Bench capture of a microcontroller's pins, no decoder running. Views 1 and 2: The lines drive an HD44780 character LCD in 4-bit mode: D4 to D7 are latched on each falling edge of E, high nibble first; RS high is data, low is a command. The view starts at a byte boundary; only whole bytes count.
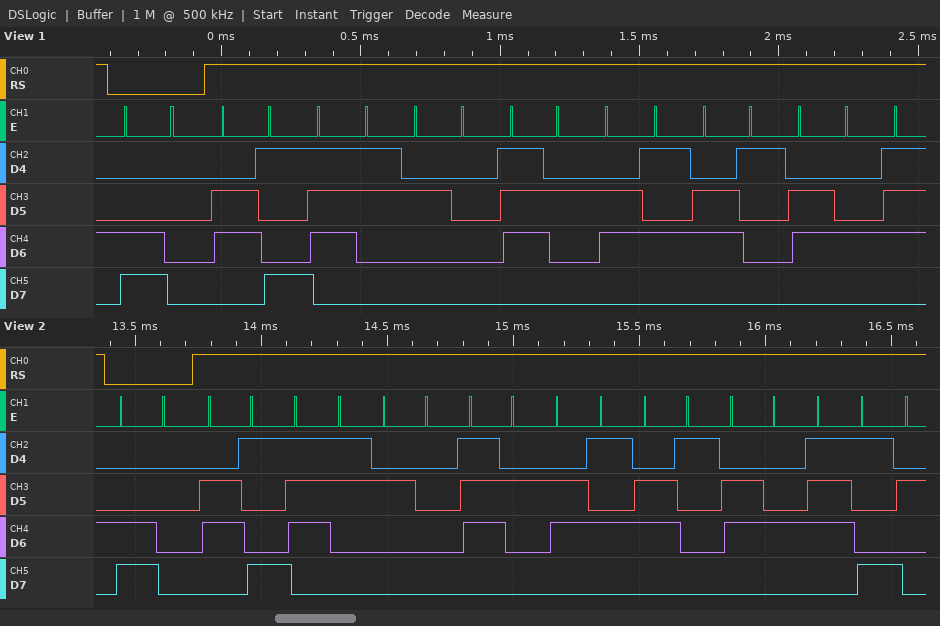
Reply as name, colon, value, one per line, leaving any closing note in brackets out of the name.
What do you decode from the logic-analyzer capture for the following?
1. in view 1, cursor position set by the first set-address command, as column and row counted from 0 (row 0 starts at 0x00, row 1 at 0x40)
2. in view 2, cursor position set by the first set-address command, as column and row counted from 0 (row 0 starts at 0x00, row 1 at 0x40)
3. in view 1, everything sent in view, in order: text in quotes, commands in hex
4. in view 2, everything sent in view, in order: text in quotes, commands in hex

in view 1, cursor position set by the first set-address command, as column and row counted from 0: column 0, row 1
in view 2, cursor position set by the first set-address command, as column and row counted from 0: column 0, row 1
in view 1, everything sent in view, in order: text in quotes, commands in hex: 0xC0 "is read"
in view 2, everything sent in view, in order: text in quotes, commands in hex: 0xC0 "is ready"
